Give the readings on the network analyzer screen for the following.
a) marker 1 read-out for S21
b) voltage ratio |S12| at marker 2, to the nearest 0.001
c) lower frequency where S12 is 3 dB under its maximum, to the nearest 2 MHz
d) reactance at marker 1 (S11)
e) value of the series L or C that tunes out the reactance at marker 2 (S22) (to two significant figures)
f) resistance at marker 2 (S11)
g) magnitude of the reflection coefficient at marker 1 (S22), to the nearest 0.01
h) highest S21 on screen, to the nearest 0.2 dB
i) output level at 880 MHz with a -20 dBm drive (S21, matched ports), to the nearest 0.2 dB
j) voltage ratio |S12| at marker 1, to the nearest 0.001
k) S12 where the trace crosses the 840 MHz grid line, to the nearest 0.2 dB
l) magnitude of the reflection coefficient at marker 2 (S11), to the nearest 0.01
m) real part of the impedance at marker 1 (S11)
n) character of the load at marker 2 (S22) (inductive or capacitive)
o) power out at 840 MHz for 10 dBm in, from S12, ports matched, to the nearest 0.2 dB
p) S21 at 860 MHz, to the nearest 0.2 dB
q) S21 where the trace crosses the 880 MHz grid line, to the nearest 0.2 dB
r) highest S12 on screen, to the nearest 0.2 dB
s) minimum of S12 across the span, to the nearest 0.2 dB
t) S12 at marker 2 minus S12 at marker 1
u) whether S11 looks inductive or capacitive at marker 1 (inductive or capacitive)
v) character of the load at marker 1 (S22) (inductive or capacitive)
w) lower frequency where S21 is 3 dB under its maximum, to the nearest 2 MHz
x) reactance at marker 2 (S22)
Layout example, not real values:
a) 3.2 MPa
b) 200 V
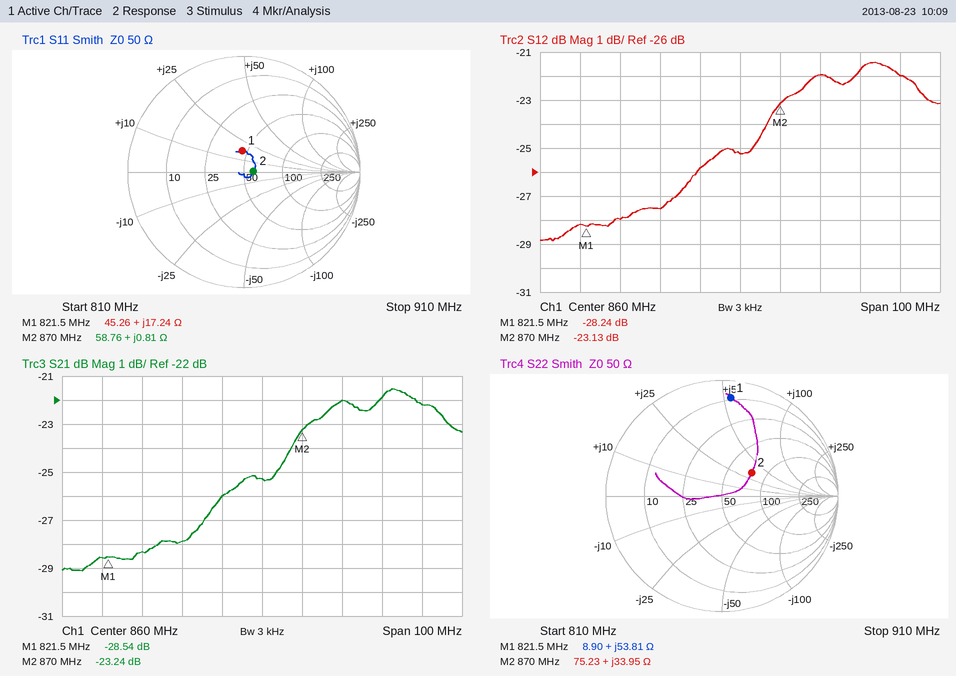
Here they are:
a) -28.54 dB
b) 0.070
c) 866 MHz
d) +17.24 Ω
e) 5.4 pF
f) 58.76 Ω
g) 0.85
h) -21.6 dB
i) -42.0 dBm
j) 0.039
k) -27.6 dB
l) 0.08
m) 45.26 Ω
n) inductive
o) -17.6 dBm
p) -25.2 dB
q) -22.0 dB
r) -21.4 dB
s) -28.8 dB
t) 5.11 dB
u) inductive
v) inductive
w) 866 MHz
x) +33.95 Ω
